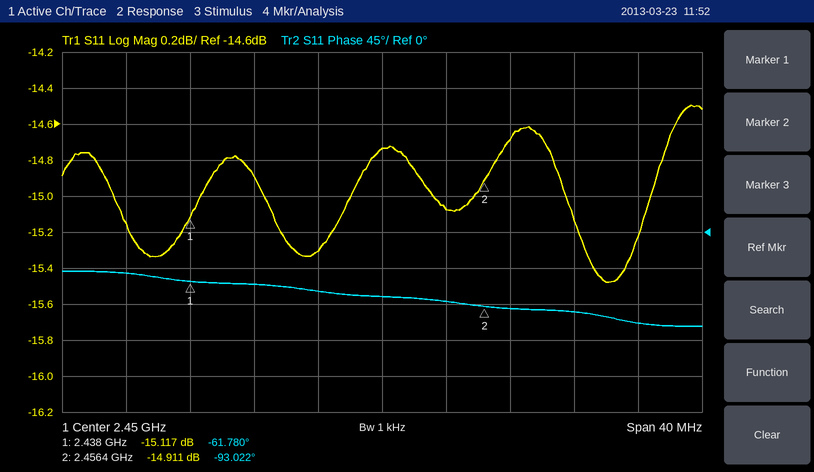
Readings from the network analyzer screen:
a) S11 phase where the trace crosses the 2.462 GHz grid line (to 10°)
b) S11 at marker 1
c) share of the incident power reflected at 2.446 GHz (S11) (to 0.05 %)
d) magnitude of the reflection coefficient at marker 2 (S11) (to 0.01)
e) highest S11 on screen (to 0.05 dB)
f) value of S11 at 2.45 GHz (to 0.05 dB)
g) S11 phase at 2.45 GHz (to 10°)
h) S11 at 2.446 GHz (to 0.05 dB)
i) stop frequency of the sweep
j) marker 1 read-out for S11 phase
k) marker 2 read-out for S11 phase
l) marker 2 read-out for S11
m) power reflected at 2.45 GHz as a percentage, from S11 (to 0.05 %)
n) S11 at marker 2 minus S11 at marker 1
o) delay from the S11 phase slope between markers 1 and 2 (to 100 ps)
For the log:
-100°
-15.117 dB
2.95 %
0.18
-14.50 dB
-14.75 dB
-80°
-15.30 dB
2.47 GHz
-61.780°
-93.022°
-14.911 dB
3.35 %
0.206 dB
4.7 ns
